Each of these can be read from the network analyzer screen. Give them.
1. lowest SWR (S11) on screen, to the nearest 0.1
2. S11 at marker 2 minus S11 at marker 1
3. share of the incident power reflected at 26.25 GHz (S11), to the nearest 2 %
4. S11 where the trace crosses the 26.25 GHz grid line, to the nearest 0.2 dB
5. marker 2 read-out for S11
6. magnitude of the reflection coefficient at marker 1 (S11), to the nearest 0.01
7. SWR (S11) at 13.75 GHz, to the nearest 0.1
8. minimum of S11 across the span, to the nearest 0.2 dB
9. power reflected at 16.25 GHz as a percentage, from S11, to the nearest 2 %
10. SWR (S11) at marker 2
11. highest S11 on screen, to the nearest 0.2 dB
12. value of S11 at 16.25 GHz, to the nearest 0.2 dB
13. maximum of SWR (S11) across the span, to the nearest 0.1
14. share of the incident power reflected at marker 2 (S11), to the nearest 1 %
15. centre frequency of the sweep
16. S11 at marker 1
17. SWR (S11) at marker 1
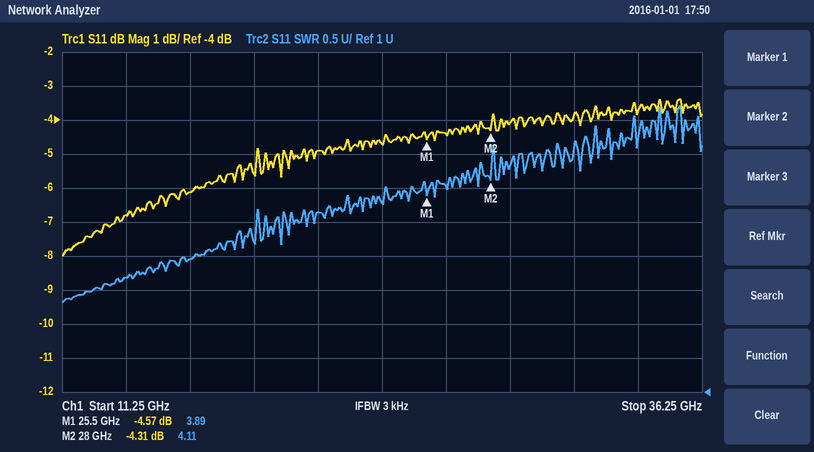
2.3
0.26 dB
36 %
-4.4 dB
-4.31 dB
0.59
2.7
-8.0 dB
24 %
4.11
-3.4 dB
-6.2 dB
5.2
37 %
23.75 GHz
-4.57 dB
3.89
